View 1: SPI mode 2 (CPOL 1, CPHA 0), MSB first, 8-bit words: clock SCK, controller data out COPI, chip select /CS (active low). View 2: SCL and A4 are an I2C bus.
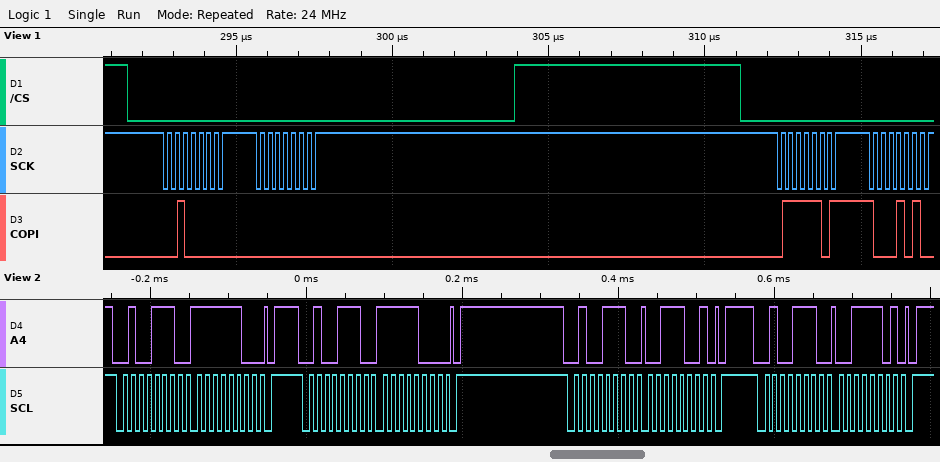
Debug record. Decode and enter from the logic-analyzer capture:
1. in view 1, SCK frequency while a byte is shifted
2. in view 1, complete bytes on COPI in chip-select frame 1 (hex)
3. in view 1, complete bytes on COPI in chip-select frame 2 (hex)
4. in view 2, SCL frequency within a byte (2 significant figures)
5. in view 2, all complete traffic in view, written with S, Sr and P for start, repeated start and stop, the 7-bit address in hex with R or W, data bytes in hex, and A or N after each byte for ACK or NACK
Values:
4 MHz
20 00
7D 8A
100 kHz
S 27W A FC A P S 27W A F8 A P S 27W A 39 A P S 27W A 3D A P
